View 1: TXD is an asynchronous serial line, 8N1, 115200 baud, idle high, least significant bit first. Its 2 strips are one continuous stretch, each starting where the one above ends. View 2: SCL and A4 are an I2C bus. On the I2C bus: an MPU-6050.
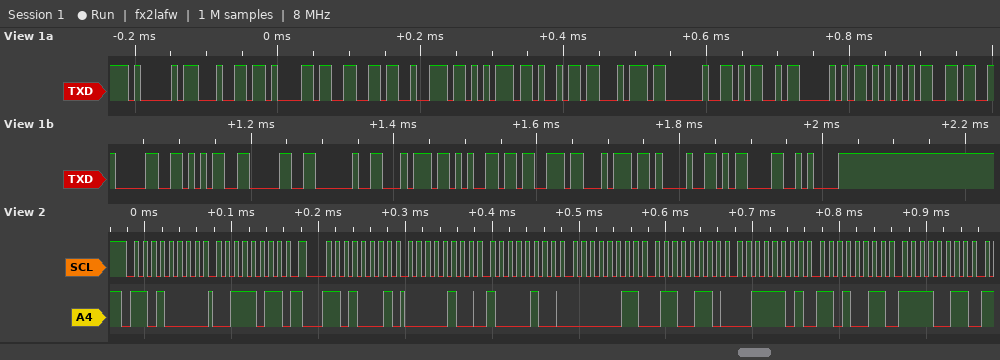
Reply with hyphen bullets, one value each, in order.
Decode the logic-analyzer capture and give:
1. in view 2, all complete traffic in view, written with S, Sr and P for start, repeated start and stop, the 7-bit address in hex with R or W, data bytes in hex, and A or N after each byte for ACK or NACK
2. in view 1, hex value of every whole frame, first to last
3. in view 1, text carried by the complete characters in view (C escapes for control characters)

- S 68W A 3B A Sr 68R A 04 A 84 A 03 A 66 A 3D A D3 A F3 A
- 0x41 0x64 0x61 0x66 0x72 0x75 0x69 0x74 0x20 0x4D 0x50 0x55 0x36 0x30 0x35 0x30 0x20 0x74 0x65 0x73 0x74 0x21 0x0D 0x0A
- "Adafruit MPU6050 test!\r\n"
